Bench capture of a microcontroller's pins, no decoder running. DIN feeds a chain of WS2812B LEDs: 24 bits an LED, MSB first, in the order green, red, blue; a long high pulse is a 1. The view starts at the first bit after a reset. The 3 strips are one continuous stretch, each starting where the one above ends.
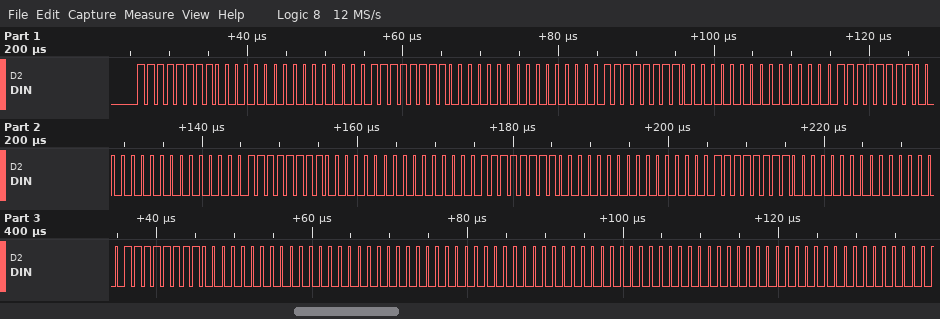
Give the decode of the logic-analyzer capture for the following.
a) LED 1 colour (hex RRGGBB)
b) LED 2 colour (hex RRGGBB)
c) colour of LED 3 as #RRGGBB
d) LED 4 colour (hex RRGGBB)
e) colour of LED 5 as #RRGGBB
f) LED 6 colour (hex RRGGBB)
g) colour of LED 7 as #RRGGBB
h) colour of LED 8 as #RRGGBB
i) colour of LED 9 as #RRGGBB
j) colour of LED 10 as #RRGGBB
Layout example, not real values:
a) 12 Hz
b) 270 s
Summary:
a) #00FF00
b) #00FF00
c) #00FF00
d) #00FF00
e) #00FF00
f) #00FF00
g) #00FF00
h) #00FF00
i) #000000
j) #000000
